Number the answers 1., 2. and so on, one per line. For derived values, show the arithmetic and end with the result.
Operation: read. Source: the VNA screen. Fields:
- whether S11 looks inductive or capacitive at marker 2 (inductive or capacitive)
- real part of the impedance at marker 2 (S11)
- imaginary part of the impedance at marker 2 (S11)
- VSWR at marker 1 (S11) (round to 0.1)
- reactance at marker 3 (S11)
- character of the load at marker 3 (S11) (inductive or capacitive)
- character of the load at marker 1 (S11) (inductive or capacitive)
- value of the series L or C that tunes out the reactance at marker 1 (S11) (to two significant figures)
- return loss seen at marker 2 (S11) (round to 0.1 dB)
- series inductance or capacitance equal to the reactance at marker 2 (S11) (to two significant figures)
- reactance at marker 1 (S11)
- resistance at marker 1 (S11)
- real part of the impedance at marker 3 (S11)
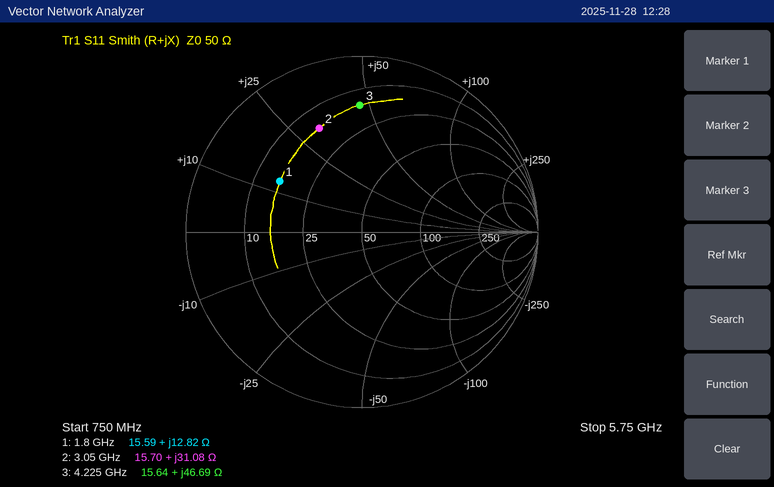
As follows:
1. inductive
2. 15.70 Ω
3. +31.08 Ω
4. 3.4
5. +46.69 Ω
6. inductive
7. inductive
8. C = 1/(2π × 1.8 GHz × 12.82 Ω) ≈ 6.9 pF
9. 3.9 dB
10. L = 31.08 Ω/(2π × 3.05 GHz) ≈ 1.6 nH
11. +12.82 Ω
12. 15.59 Ω
13. 15.64 Ω
